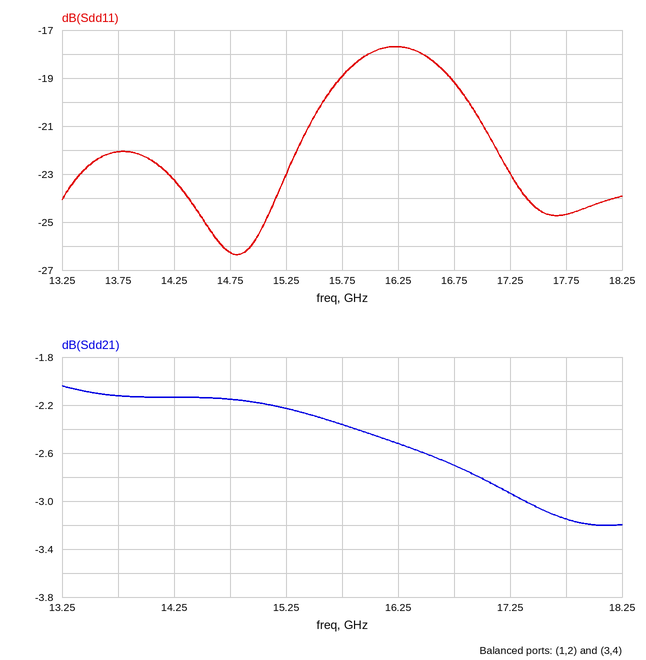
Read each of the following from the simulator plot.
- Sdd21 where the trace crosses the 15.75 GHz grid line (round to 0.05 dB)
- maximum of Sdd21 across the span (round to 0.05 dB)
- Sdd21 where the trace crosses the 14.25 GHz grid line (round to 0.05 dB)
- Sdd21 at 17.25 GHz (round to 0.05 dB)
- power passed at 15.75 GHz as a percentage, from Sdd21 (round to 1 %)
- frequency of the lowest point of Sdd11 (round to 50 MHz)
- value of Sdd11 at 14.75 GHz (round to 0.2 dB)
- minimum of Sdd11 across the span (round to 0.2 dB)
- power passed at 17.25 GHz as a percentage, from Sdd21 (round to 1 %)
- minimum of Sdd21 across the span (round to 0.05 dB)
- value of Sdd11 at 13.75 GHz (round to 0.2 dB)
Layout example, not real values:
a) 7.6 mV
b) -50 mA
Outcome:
a) -2.35 dB
b) -2.05 dB
c) -2.15 dB
d) -2.95 dB
e) 58 %
f) 14.80 GHz
g) -26.2 dB
h) -26.4 dB
i) 51 %
j) -3.20 dB
k) -22.0 dB
